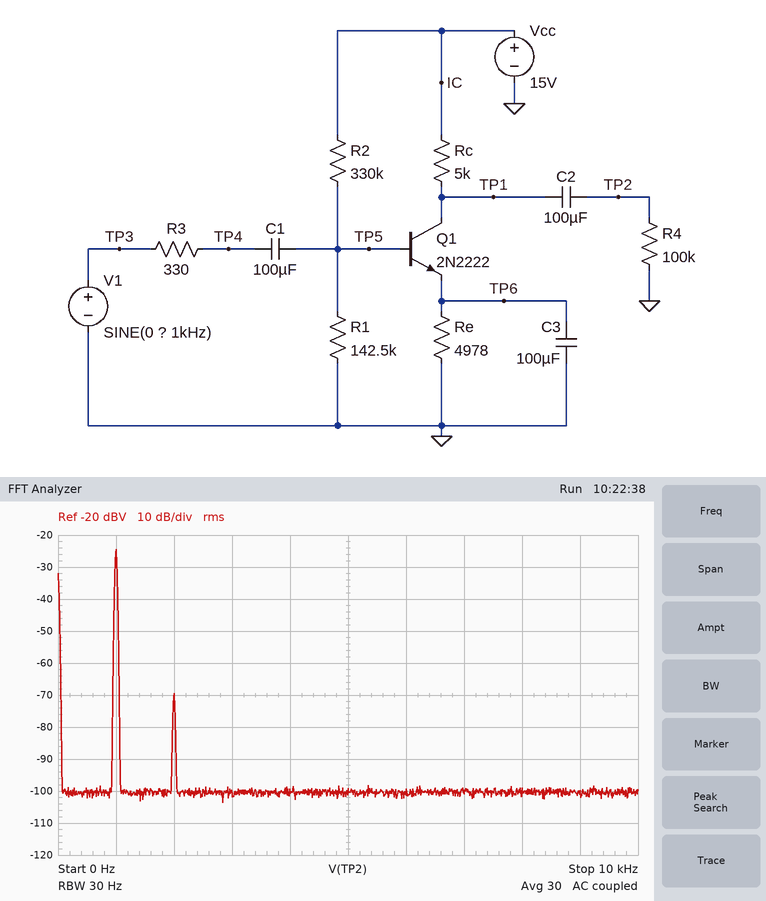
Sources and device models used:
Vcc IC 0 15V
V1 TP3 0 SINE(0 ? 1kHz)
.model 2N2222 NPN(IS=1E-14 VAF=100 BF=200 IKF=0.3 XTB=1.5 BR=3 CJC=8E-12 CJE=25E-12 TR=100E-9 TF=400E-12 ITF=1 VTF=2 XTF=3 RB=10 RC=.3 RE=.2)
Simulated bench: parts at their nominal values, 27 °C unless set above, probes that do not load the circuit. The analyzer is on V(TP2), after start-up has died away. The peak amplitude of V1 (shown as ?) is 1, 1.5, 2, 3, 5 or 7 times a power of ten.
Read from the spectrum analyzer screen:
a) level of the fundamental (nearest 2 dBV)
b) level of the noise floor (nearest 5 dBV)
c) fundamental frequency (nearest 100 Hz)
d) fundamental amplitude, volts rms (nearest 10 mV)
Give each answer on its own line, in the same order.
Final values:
-24 dBV
-100 dBV
1.0 kHz
60 mV
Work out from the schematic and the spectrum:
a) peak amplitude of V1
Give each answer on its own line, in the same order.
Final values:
700 µV
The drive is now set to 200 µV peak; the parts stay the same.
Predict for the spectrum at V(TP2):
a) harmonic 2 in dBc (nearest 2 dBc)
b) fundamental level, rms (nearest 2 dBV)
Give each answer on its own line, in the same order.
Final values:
-56 dBc
-36 dBV
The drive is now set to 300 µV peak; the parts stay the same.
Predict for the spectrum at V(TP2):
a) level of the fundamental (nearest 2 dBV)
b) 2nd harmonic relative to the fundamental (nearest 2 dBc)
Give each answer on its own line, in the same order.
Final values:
-32 dBV
-52 dBc
